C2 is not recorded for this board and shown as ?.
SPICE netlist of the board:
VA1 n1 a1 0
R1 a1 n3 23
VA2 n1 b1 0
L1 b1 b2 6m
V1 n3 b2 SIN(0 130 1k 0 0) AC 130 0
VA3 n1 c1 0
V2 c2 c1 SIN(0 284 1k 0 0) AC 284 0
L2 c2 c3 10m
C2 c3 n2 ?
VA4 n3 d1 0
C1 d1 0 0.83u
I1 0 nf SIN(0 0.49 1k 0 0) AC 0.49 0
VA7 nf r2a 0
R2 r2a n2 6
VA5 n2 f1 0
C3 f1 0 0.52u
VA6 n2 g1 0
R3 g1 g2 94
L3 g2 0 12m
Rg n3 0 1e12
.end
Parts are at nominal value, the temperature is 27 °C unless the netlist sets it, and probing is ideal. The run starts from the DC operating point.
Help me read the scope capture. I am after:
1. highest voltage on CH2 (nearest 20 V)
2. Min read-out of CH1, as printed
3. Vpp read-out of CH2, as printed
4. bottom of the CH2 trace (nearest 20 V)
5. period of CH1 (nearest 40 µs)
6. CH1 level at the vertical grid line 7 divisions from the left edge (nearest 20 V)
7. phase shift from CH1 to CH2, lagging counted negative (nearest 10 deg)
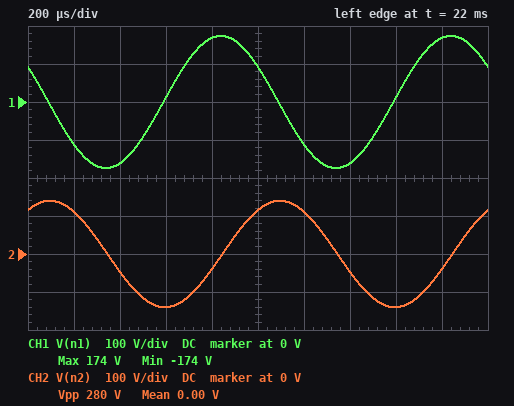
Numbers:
140 V
-174 V
280 V
-140 V
1.00 ms
-160 V
-90 deg
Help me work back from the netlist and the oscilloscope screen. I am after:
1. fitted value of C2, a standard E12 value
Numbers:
1 µF
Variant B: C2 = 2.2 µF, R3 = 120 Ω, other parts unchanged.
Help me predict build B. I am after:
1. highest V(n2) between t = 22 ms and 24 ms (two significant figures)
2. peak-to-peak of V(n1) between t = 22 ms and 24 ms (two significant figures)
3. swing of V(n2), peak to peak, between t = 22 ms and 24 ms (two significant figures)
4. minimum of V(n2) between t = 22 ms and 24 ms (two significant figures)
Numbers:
170 V
370 V
340 V
-170 V
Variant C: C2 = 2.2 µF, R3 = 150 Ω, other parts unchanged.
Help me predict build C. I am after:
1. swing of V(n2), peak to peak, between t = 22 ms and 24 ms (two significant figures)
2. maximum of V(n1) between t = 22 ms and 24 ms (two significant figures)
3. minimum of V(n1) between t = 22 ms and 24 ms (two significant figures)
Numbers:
330 V
160 V
-160 V
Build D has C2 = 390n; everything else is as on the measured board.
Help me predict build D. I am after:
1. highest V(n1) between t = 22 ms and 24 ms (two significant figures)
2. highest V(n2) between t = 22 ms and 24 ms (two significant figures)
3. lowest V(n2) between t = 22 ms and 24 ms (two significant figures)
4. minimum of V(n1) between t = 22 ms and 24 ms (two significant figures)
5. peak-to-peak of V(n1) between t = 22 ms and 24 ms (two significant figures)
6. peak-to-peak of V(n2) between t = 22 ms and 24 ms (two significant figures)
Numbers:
120 V
95 V
-95 V
-120 V
230 V
190 V
